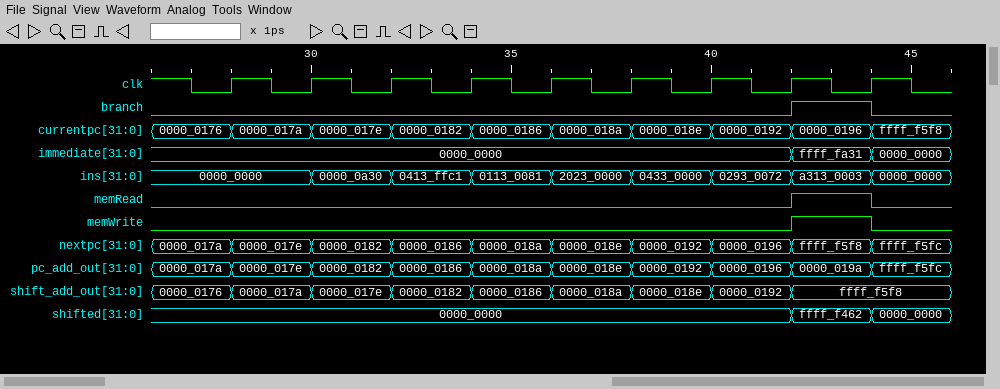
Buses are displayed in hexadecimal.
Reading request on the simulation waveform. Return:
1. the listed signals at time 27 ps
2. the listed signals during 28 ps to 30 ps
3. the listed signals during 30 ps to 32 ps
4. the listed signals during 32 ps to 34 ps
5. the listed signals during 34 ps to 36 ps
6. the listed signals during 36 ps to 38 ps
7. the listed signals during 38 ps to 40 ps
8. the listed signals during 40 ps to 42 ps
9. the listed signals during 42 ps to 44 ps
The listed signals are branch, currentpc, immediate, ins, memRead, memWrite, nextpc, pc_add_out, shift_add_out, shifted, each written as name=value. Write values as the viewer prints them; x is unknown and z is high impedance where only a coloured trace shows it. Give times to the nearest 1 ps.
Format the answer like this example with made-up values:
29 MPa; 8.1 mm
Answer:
branch=0, currentpc=0000_0176, immediate=0000_0000, ins=0000_0000, memRead=0, memWrite=0, nextpc=0000_017a, pc_add_out=0000_017a, shift_add_out=0000_0176, shifted=0000_0000; branch=0, currentpc=0000_017a, immediate=0000_0000, ins=0000_0000, memRead=0, memWrite=0, nextpc=0000_017e, pc_add_out=0000_017e, shift_add_out=0000_017a, shifted=0000_0000; branch=0, currentpc=0000_017e, immediate=0000_0000, ins=0000_0a30, memRead=0, memWrite=0, nextpc=0000_0182, pc_add_out=0000_0182, shift_add_out=0000_017e, shifted=0000_0000; branch=0, currentpc=0000_0182, immediate=0000_0000, ins=0413_ffc1, memRead=0, memWrite=0, nextpc=0000_0186, pc_add_out=0000_0186, shift_add_out=0000_0182, shifted=0000_0000; branch=0, currentpc=0000_0186, immediate=0000_0000, ins=0113_0081, memRead=0, memWrite=0, nextpc=0000_018a, pc_add_out=0000_018a, shift_add_out=0000_0186, shifted=0000_0000; branch=0, currentpc=0000_018a, immediate=0000_0000, ins=2023_0000, memRead=0, memWrite=0, nextpc=0000_018e, pc_add_out=0000_018e, shift_add_out=0000_018a, shifted=0000_0000; branch=0, currentpc=0000_018e, immediate=0000_0000, ins=0433_0000, memRead=0, memWrite=0, nextpc=0000_0192, pc_add_out=0000_0192, shift_add_out=0000_018e, shifted=0000_0000; branch=0, currentpc=0000_0192, immediate=0000_0000, ins=0293_0072, memRead=0, memWrite=0, nextpc=0000_0196, pc_add_out=0000_0196, shift_add_out=0000_0192, shifted=0000_0000; branch=1, currentpc=0000_0196, immediate=ffff_fa31, ins=a313_0003, memRead=1, memWrite=1, nextpc=ffff_f5f8, pc_add_out=0000_019a, shift_add_out=ffff_f5f8, shifted=ffff_f462
